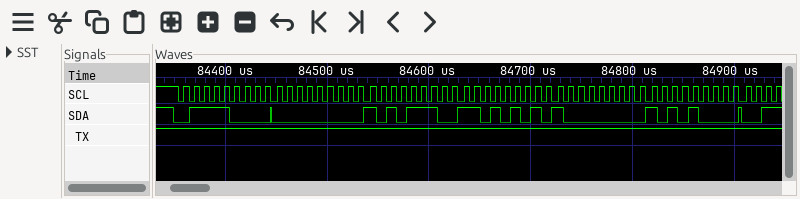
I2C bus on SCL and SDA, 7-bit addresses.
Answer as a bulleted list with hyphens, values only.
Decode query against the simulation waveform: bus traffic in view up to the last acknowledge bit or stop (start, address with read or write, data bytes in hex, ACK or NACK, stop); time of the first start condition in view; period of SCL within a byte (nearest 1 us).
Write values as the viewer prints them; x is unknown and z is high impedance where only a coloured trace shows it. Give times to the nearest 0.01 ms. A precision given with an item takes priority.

- start, address 3C write ACK, 00 ACK, AE ACK, D5 ACK, 80 ACK, A8 ACK
- 84.35 ms
- 10 us
